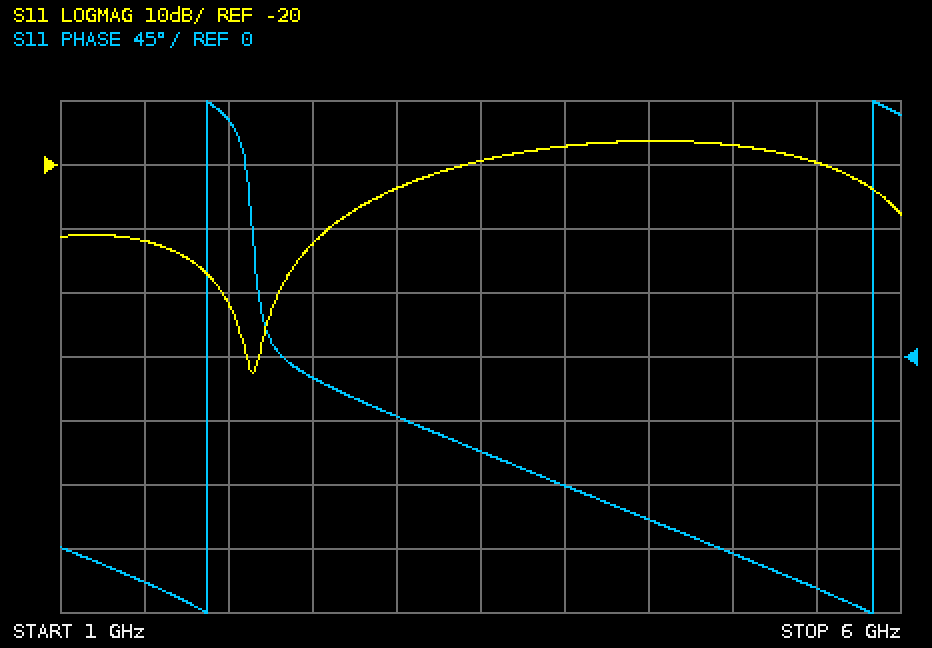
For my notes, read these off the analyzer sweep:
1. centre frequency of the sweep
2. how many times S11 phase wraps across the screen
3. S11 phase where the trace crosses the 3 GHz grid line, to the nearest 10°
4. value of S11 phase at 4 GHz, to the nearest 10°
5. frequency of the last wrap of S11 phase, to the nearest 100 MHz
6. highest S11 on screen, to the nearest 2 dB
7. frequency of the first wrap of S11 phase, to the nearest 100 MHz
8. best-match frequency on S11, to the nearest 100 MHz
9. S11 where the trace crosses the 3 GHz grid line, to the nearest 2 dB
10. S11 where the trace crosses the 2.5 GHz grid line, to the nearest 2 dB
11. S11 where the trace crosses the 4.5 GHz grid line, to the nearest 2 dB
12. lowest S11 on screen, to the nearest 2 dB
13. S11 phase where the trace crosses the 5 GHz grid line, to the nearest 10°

3.5 GHz
2
-40°
-90°
5.8 GHz
-16 dB
1.9 GHz
2.1 GHz
-24 dB
-32 dB
-16 dB
-52 dB
-140°
